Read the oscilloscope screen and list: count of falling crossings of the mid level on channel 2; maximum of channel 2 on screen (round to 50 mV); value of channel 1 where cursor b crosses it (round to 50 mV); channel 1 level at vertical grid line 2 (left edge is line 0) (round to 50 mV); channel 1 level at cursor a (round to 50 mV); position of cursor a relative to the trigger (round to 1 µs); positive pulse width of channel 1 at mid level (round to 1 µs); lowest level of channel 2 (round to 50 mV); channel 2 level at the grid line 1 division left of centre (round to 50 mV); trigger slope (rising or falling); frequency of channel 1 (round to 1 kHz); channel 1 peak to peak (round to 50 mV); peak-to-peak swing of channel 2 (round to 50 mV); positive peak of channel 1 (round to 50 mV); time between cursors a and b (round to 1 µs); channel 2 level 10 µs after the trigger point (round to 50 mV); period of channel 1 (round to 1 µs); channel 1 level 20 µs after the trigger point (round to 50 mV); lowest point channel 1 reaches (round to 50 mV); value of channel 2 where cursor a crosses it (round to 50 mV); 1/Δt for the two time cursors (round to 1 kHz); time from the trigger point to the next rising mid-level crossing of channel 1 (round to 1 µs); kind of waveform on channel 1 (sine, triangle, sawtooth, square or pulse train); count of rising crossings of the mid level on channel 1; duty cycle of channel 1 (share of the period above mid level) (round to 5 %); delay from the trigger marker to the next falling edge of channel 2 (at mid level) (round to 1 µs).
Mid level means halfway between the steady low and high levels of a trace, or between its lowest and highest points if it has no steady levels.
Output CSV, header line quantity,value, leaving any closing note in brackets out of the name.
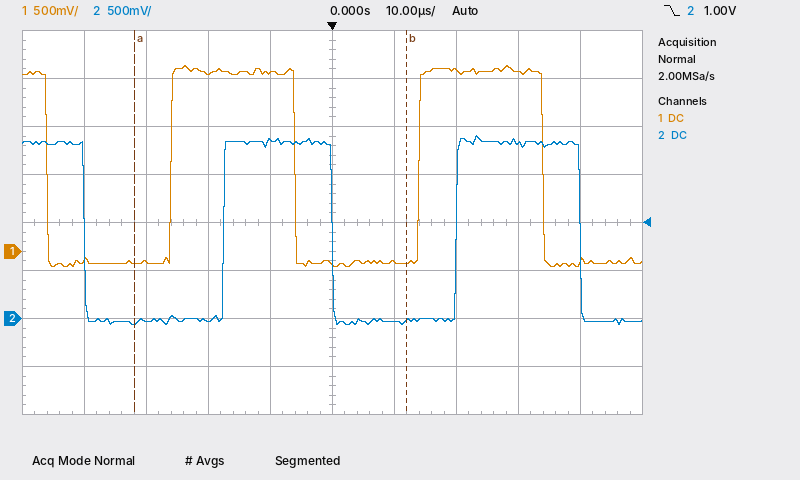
quantity,value
count of falling crossings of the mid level on channel 2,3
maximum of channel 2 on screen,1.90 V
value of channel 1 where cursor b crosses it,-100 mV
channel 1 level at vertical grid line 2 (left edge is line 0),-100 mV
channel 1 level at cursor a,-100 mV
position of cursor a relative to the trigger,-32 µs
positive pulse width of channel 1 at mid level,20 µs
lowest level of channel 2,-50 mV
channel 2 level at the grid line 1 division left of centre,1.85 V
trigger slope,falling
frequency of channel 1,25 kHz
channel 1 peak to peak,2.10 V
peak-to-peak swing of channel 2,1.95 V
positive peak of channel 1,1.95 V
time between cursors a and b,44 µs
channel 2 level 10 µs after the trigger point,-50 mV
period of channel 1,40 µs
channel 1 level 20 µs after the trigger point,1.90 V
lowest point channel 1 reaches,-150 mV
value of channel 2 where cursor a crosses it,-50 mV
1/Δt for the two time cursors,23 kHz
time from the trigger point to the next rising mid-level crossing of channel 1,14 µs
kind of waveform on channel 1,square
count of rising crossings of the mid level on channel 1,2
duty cycle of channel 1 (share of the period above mid level),50 %
delay from the trigger marker to the next falling edge of channel 2 (at mid level),40 µs
